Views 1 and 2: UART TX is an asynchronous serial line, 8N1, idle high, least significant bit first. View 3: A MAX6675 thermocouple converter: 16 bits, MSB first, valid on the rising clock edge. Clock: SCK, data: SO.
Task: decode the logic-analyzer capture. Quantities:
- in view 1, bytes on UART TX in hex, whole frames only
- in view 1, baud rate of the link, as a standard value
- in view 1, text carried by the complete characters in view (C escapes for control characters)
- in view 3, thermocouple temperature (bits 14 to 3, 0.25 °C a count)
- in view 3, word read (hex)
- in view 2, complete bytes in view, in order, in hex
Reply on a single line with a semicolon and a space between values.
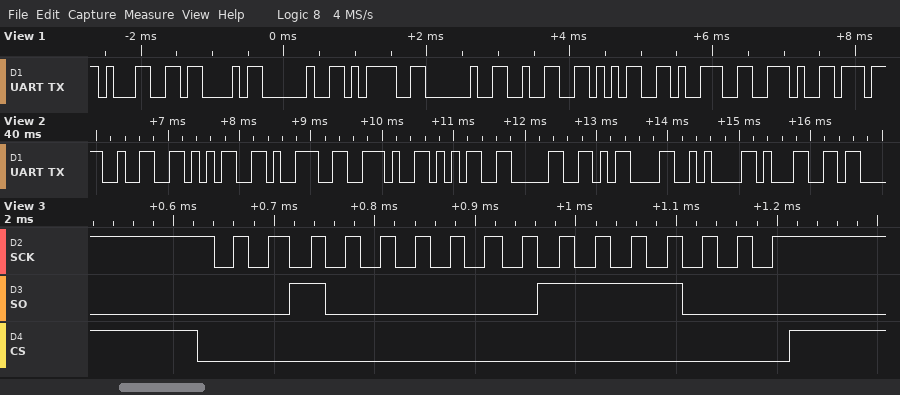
31 43 20 3D 20 32 35 39 2E; 9600 baud; "1C = 259."; 259.75 °C; 0x2078; 0x32 0x35 0x39 0x2E 0x35 0x30 0x0D 0x0A 0x31
